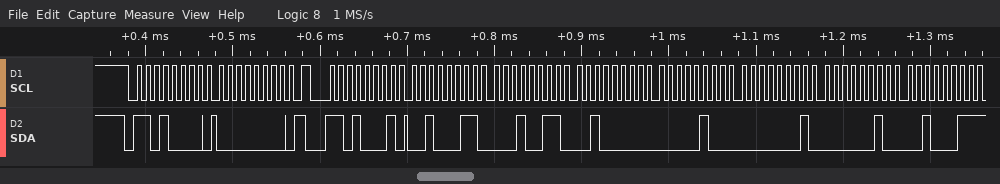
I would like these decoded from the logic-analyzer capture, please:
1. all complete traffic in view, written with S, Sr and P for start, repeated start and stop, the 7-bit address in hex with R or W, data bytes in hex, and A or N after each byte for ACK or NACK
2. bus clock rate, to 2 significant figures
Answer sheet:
S 68W A 00 A Sr 68R A 23 A 13 A 20 A 04 A 01 A 02 A 23 N
100 kHz
